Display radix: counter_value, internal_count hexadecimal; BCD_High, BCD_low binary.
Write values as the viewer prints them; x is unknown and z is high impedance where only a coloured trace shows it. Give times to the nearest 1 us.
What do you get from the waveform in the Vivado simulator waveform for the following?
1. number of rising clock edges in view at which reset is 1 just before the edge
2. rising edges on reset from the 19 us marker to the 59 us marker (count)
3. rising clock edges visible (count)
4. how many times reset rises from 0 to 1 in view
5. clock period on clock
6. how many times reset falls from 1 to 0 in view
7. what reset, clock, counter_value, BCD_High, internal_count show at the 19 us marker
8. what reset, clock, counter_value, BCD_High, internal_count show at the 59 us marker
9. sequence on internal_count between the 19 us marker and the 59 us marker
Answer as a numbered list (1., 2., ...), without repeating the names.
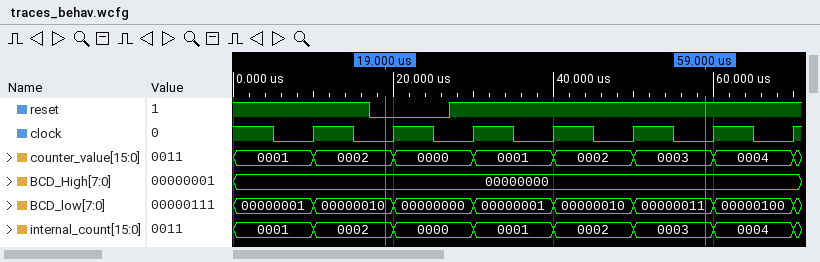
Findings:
1. 6
2. 1
3. 7
4. 1
5. 10 us
6. 1
7. reset=0, clock=0, counter_value=0002, BCD_High=00000000, internal_count=0002
8. reset=1, clock=0, counter_value=0003, BCD_High=00000000, internal_count=0003
9. 0002, 0000, 0001, 0002, 0003
